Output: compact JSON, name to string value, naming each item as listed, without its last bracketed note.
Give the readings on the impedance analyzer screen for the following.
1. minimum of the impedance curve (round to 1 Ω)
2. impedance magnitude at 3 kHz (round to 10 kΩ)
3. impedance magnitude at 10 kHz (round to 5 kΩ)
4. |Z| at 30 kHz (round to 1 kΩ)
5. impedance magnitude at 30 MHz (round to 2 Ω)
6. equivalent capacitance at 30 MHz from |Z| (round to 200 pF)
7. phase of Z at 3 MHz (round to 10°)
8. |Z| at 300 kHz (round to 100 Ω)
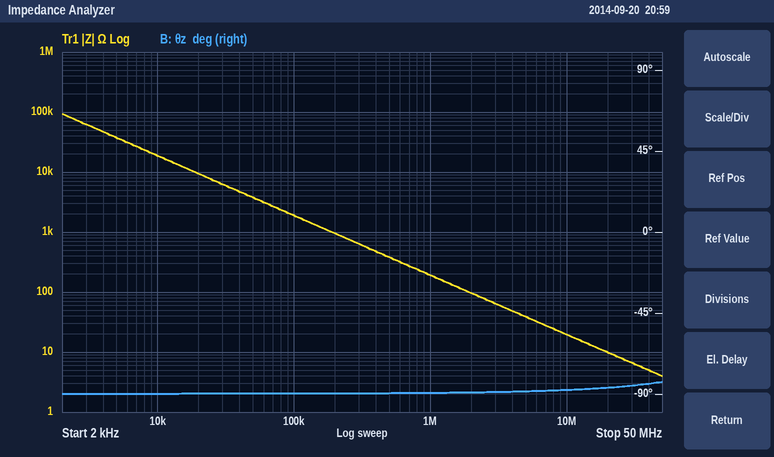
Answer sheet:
{"minimum of the impedance curve": "4 Ω", "impedance magnitude at 3 kHz": "60 kΩ", "impedance magnitude at 10 kHz": "20 kΩ", "|Z| at 30 kHz": "6 kΩ", "impedance magnitude at 30 MHz": "6 Ω", "equivalent capacitance at 30 MHz from |Z|": "800 pF", "phase of Z at 3 MHz": "-90°", "|Z| at 300 kHz": "600 Ω"}
